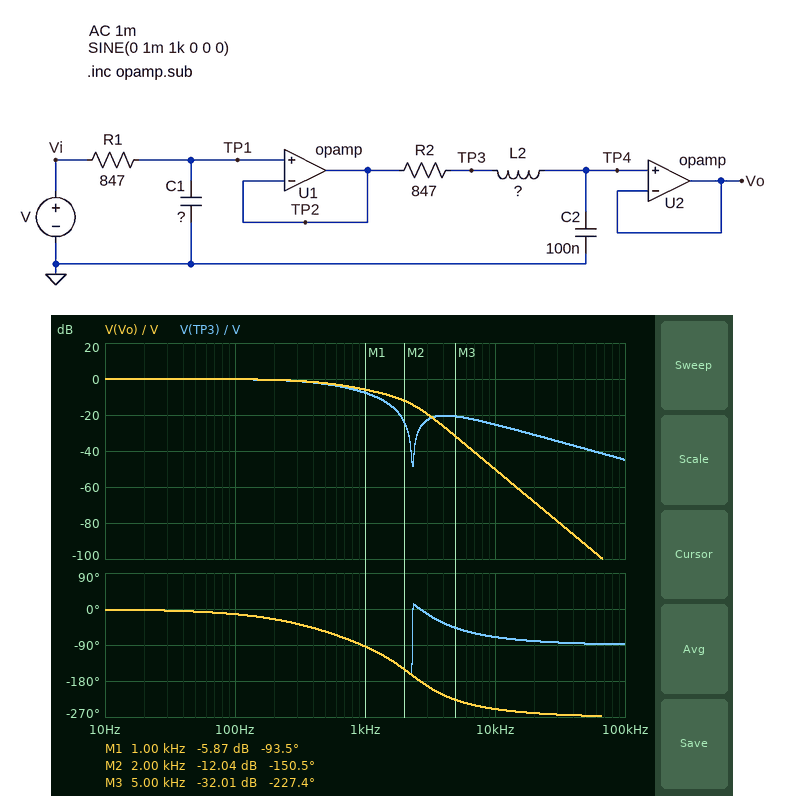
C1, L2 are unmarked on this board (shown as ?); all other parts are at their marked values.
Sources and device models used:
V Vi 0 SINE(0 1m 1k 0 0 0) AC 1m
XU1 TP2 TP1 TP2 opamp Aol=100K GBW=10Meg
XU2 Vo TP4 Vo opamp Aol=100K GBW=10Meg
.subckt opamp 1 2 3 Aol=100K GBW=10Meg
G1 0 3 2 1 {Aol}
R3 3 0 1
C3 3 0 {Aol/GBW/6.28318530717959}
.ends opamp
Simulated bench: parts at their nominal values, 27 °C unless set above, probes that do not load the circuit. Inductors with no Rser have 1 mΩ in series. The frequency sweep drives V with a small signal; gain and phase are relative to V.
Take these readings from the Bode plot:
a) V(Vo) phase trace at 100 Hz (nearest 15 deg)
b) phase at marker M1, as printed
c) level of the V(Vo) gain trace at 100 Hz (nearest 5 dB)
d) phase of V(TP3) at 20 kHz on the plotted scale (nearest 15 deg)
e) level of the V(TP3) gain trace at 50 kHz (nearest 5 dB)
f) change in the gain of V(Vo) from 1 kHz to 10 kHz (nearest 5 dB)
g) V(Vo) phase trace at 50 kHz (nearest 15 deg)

-15 deg
-93.5 deg
0 dB
-75 deg
-40 dB
-45 dB
-270 deg
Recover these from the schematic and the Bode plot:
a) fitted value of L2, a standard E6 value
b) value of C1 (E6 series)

47 mH
330 nF
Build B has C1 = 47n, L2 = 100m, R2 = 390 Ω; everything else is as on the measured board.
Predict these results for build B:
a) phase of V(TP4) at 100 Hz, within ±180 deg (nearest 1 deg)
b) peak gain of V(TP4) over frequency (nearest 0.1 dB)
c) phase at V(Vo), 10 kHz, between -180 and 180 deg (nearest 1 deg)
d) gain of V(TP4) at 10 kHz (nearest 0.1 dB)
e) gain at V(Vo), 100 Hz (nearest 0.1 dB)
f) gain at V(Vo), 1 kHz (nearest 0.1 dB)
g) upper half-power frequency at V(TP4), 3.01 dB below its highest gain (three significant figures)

-3 deg
7.8 dB
115 deg
-40.3 dB
0 dB
3.4 dB
1.81 kHz
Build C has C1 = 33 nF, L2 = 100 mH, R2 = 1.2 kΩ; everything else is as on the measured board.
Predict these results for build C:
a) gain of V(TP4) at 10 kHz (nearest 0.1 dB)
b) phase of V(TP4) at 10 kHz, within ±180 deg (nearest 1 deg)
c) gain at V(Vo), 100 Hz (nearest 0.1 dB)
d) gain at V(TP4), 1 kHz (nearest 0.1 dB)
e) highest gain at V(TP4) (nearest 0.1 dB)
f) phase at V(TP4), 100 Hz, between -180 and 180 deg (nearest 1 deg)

-38.0 dB
131 deg
0 dB
0.2 dB
0.3 dB
-5 deg
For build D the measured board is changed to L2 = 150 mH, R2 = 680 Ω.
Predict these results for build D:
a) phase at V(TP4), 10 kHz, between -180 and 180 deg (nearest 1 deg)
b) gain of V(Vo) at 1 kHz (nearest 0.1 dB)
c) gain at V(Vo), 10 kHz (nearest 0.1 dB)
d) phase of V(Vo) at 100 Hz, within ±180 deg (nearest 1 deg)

97 deg
-1.5 dB
-60.2 dB
-12 deg
